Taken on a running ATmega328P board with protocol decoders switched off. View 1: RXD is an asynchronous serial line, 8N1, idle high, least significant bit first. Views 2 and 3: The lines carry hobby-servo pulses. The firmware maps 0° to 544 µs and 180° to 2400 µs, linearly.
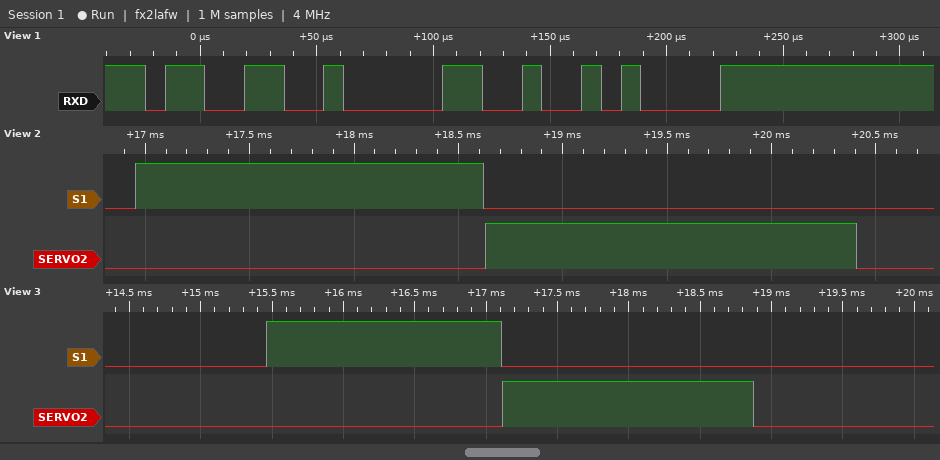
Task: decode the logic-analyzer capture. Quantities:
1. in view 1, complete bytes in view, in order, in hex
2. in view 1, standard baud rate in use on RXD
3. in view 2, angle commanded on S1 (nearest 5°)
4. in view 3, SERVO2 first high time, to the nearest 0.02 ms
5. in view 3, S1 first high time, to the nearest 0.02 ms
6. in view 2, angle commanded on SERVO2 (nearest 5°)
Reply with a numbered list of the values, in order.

1. 0x33 0x30 0x0A
2. 115200 baud
3. 110°
4. 1.76 ms
5. 1.64 ms
6. 120°
